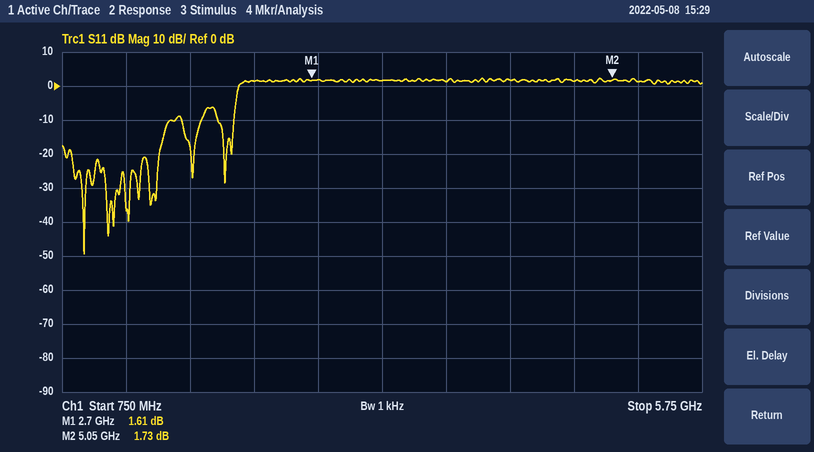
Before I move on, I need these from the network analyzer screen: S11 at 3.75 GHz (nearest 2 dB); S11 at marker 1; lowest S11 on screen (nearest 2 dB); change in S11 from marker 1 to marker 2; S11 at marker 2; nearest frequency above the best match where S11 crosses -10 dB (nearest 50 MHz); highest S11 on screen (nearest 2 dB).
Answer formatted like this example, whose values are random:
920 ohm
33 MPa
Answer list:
2 dB
1.61 dB
-50 dB
0.12 dB
1.73 dB
1.65 GHz
2 dB
